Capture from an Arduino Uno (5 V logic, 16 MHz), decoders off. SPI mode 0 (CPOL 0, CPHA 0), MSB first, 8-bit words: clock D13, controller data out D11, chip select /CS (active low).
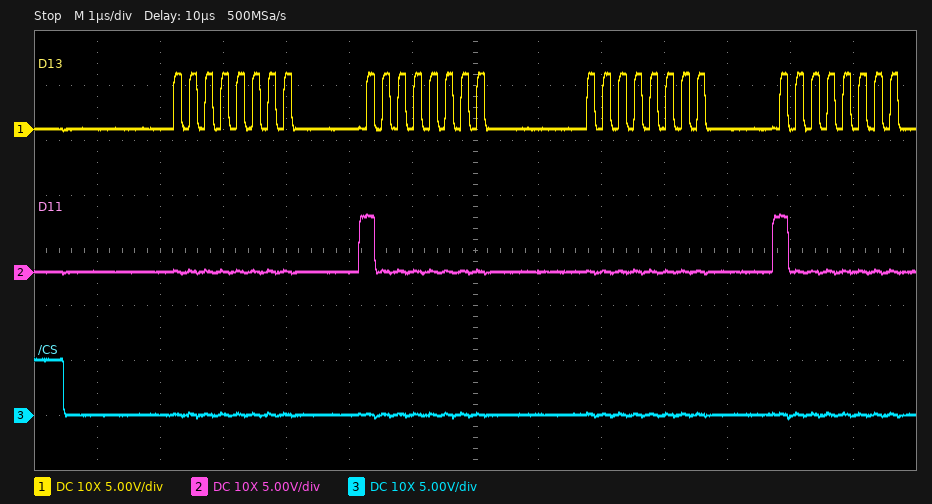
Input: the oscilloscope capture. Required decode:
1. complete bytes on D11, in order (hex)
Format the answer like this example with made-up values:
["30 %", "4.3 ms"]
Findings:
["00 80 00 80"]
